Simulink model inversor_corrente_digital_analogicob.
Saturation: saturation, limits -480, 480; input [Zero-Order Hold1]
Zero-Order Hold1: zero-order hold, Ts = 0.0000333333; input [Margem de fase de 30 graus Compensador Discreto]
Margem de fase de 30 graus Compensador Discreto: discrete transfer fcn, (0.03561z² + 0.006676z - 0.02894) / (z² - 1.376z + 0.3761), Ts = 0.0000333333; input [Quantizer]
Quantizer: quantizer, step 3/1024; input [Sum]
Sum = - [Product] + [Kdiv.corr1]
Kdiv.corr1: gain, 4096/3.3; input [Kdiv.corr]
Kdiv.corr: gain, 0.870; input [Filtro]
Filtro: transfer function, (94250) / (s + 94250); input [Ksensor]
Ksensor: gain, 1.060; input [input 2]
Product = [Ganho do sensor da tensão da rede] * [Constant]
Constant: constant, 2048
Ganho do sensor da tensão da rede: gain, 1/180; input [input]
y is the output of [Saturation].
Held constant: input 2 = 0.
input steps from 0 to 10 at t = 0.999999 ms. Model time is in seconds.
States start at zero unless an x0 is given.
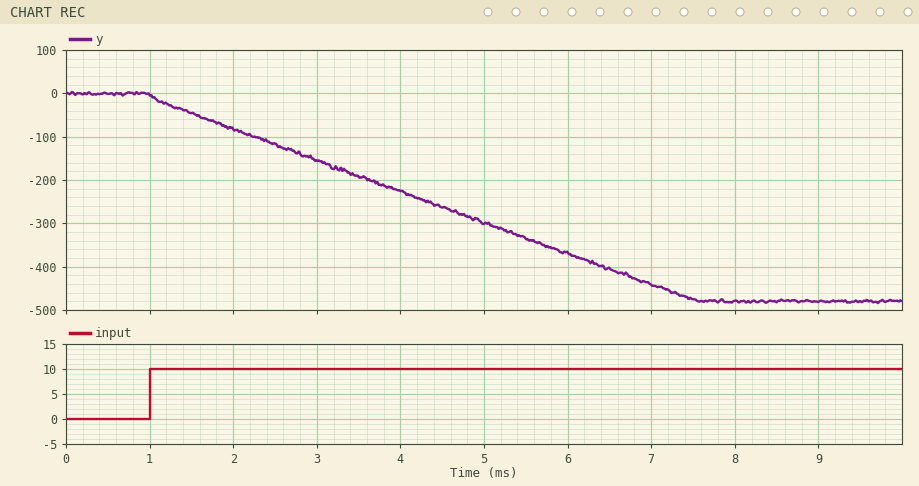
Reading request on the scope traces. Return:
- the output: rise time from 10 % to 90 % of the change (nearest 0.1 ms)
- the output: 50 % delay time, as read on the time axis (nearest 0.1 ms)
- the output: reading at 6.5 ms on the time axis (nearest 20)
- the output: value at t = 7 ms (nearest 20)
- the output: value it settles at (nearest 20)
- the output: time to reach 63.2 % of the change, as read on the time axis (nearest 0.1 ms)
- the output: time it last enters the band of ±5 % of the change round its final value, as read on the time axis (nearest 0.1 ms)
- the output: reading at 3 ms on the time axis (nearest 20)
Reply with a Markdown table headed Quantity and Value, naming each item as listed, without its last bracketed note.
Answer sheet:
| Quantity | Value |
|---|---|
| the output: rise time from 10 % to 90 % of the change | 5.3 ms |
| the output: 50 % delay time, as read on the time axis | 4.2 ms |
| the output: reading at 6.5 ms on the time axis | -400 |
| the output: value at t = 7 ms | -440 |
| the output: value it settles at | -480 |
| the output: time to reach 63.2 % of the change, as read on the time axis | 5.1 ms |
| the output: time it last enters the band of ±5 % of the change round its final value, as read on the time axis | 7.2 ms |
| the output: reading at 3 ms on the time axis | -160 |
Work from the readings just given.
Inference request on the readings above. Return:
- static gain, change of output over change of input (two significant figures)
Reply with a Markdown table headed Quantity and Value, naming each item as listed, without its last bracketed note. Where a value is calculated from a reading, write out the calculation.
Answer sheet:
| Quantity | Value |
|---|---|
| static gain, change of output over change of input | (-480 - 0) / (10 - 0) = -48 |
